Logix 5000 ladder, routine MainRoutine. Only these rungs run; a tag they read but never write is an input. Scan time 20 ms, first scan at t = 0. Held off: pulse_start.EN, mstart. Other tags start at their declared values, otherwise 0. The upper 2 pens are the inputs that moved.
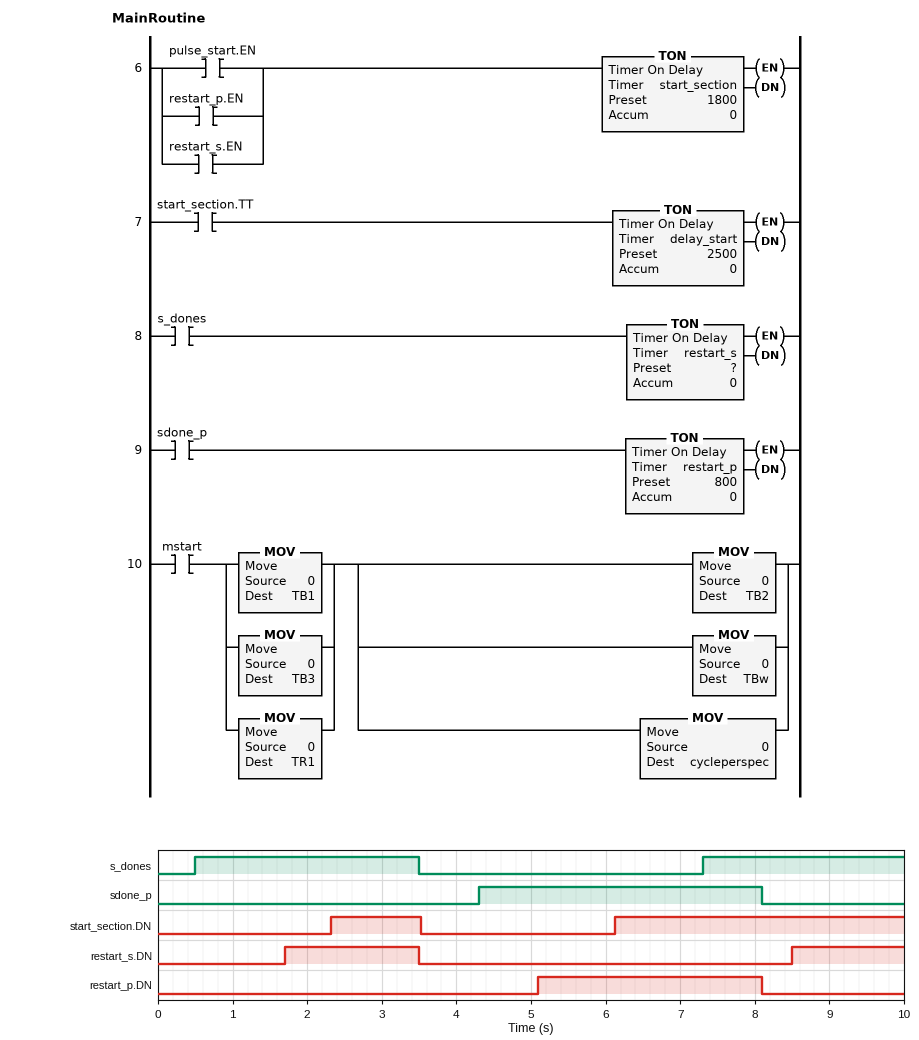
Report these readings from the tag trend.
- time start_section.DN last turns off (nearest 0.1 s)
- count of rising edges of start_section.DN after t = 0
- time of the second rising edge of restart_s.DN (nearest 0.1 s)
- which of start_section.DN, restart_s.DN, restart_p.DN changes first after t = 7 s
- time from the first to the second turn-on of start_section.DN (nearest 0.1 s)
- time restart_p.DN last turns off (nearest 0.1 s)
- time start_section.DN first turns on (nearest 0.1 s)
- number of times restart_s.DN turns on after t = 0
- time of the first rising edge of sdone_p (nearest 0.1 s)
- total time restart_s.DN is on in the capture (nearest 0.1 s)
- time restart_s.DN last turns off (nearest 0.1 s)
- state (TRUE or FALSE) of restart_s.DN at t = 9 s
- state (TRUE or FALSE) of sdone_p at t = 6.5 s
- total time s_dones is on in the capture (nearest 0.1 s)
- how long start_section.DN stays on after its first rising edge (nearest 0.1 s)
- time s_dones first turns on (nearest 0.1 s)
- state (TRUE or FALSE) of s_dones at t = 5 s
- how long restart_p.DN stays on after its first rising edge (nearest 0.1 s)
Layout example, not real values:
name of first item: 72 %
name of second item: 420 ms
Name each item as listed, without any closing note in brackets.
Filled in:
time start_section.DN last turns off: 3.5 s
count of rising edges of start_section.DN after t = 0: 2
time of the second rising edge of restart_s.DN: 8.5 s
which of start_section.DN, restart_s.DN, restart_p.DN changes first after t = 7 s: restart_p.DN
time from the first to the second turn-on of start_section.DN: 3.8 s
time restart_p.DN last turns off: 8.1 s
time start_section.DN first turns on: 2.3 s
number of times restart_s.DN turns on after t = 0: 2
time of the first rising edge of sdone_p: 4.3 s
total time restart_s.DN is on in the capture: 3.3 s
time restart_s.DN last turns off: 3.5 s
state (TRUE or FALSE) of restart_s.DN at t = 9 s: TRUE
state (TRUE or FALSE) of sdone_p at t = 6.5 s: TRUE
total time s_dones is on in the capture: 5.7 s
how long start_section.DN stays on after its first rising edge: 1.2 s
time s_dones first turns on: 0.5 s
state (TRUE or FALSE) of s_dones at t = 5 s: FALSE
how long restart_p.DN stays on after its first rising edge: 3.0 s
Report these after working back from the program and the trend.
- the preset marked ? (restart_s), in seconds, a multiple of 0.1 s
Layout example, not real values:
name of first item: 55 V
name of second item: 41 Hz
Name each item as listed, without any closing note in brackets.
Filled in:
the preset marked ? (restart_s), in seconds, a multiple of 0.1 s: 1.2 s
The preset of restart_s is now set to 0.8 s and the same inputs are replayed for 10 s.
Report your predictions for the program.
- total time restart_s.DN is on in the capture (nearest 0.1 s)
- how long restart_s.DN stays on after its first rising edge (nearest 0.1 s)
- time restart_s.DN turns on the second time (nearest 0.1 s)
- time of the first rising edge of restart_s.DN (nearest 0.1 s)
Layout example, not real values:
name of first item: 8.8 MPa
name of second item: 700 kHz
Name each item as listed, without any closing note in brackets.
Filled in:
total time restart_s.DN is on in the capture: 4.1 s
how long restart_s.DN stays on after its first rising edge: 2.2 s
time restart_s.DN turns on the second time: 8.1 s
time of the first rising edge of restart_s.DN: 1.3 s
